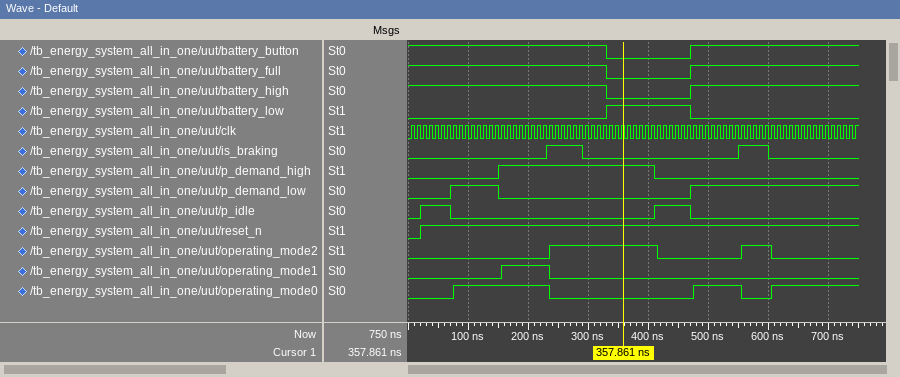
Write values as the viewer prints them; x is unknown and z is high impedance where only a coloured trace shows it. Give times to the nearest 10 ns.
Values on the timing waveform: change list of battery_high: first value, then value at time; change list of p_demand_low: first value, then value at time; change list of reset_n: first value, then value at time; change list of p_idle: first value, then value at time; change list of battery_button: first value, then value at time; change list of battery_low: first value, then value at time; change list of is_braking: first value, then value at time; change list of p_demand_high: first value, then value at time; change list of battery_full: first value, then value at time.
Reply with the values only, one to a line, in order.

1, 0 at 330 ns, 1 at 470 ns
0, 1 at 70 ns, 0 at 150 ns, 1 at 470 ns
0, 1 at 20 ns
0, 1 at 20 ns, 0 at 70 ns, 1 at 410 ns, 0 at 470 ns
1, 0 at 330 ns, 1 at 470 ns
0, 1 at 330 ns, 0 at 470 ns
0, 1 at 230 ns, 0 at 290 ns, 1 at 550 ns, 0 at 600 ns
0, 1 at 150 ns, 0 at 410 ns
1, 0 at 330 ns, 1 at 470 ns
